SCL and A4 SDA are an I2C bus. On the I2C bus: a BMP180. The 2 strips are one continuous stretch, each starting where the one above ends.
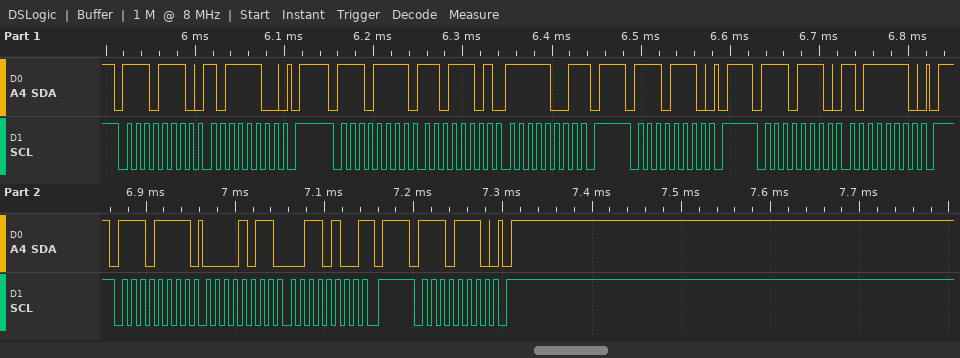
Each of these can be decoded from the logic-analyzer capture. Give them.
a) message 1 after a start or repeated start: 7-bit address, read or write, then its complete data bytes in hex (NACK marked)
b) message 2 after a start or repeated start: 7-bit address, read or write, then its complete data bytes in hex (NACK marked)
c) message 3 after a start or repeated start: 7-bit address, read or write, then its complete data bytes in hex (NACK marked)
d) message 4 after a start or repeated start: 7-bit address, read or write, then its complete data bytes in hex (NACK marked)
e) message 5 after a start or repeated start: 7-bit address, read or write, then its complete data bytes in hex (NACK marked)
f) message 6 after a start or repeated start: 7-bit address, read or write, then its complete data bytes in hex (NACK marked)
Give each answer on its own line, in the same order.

0x77 write: BC
0x77 read: DD F9 NACK
0x77 write
0x77 write: BE
0x77 read: 0B 34 NACK
0x77 write
